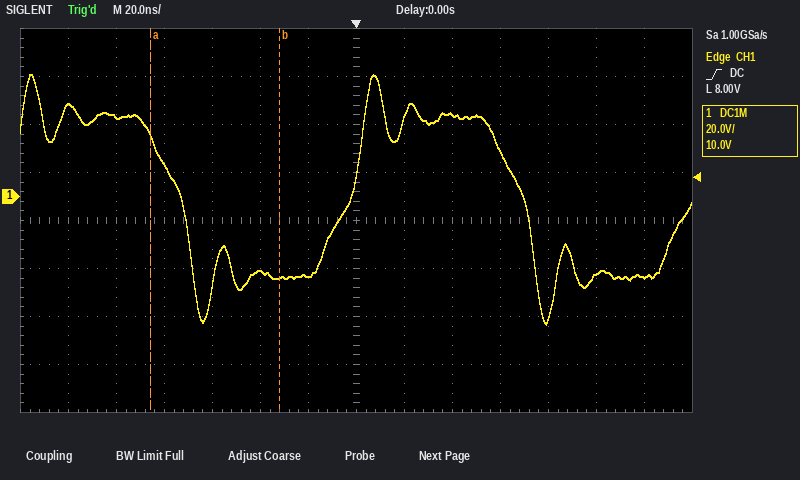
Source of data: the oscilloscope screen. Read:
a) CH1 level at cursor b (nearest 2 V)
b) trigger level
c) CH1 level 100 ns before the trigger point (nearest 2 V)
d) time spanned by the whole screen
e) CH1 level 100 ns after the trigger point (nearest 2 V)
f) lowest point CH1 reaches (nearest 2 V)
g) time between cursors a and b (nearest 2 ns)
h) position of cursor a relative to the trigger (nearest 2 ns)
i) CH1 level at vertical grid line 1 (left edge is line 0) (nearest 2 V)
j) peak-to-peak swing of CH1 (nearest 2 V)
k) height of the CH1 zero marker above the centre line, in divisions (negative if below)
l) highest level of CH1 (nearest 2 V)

-34 V
8.00 V
34 V
280 ns
-32 V
-54 V
54 ns
-86 ns
38 V
104 V
+0.5 div
50 V
